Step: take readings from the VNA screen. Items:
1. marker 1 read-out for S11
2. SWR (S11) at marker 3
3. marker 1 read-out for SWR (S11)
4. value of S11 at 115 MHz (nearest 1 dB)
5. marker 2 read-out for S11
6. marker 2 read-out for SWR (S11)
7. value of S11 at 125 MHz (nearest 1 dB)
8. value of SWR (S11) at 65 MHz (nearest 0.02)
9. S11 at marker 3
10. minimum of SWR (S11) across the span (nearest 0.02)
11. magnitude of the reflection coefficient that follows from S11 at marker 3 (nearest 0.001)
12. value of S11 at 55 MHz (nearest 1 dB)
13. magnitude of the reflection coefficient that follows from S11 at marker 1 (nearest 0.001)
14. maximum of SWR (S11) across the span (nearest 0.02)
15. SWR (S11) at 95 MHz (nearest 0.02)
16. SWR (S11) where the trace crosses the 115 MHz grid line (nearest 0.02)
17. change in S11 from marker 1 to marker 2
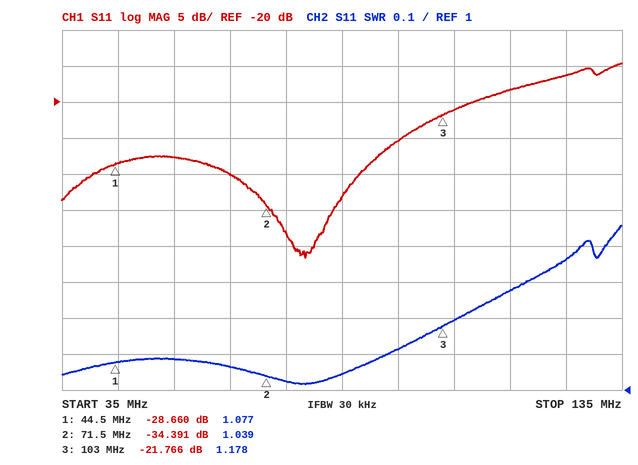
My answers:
-28.660 dB
1.178
1.077
-18 dB
-34.391 dB
1.039
-16 dB
1.06
-21.766 dB
1.02
0.082
-28 dB
0.037
1.46
1.12
1.28
-5.731 dB
